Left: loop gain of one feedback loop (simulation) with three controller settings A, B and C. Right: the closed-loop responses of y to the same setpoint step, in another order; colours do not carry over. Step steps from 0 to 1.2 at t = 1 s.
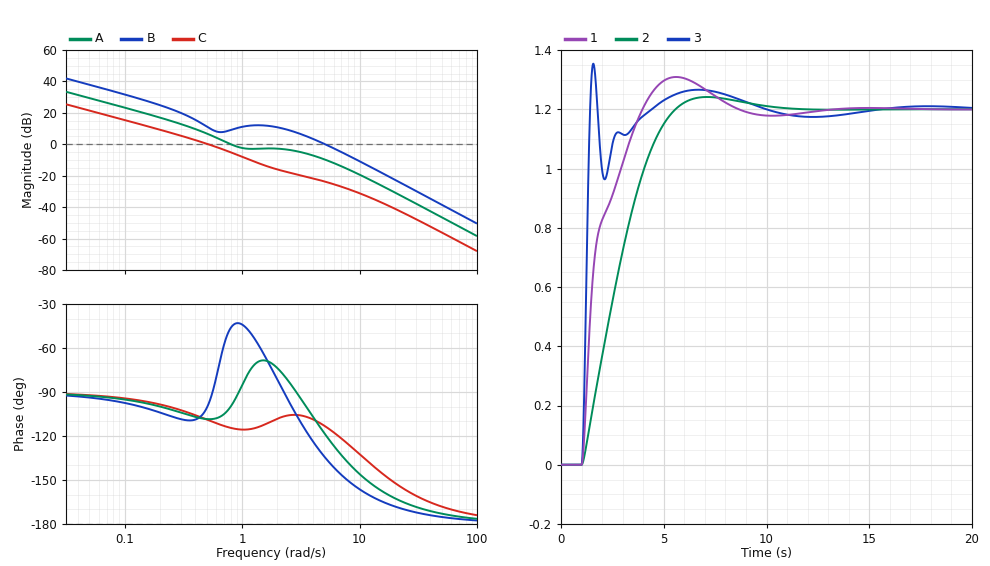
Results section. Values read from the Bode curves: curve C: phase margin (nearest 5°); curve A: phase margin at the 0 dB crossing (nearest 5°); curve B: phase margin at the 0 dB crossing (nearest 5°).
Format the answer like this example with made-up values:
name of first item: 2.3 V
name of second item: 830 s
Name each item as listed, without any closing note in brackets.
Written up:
curve C: phase margin: 70°
curve A: phase margin at the 0 dB crossing: 80°
curve B: phase margin at the 0 dB crossing: 45°
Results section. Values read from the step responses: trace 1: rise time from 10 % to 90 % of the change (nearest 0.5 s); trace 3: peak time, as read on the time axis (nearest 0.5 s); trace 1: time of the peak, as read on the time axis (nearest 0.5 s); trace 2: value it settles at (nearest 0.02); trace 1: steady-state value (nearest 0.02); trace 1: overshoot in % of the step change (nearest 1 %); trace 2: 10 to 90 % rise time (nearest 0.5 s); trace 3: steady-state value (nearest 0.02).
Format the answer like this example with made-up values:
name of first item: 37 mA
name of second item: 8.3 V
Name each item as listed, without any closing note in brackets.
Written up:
trace 1: rise time from 10 % to 90 % of the change: 2.0 s
trace 3: peak time, as read on the time axis: 1.5 s
trace 1: time of the peak, as read on the time axis: 5.5 s
trace 2: value it settles at: 1.20
trace 1: steady-state value: 1.20
trace 1: overshoot in % of the step change: 9 %
trace 2: 10 to 90 % rise time: 3.0 s
trace 3: steady-state value: 1.20
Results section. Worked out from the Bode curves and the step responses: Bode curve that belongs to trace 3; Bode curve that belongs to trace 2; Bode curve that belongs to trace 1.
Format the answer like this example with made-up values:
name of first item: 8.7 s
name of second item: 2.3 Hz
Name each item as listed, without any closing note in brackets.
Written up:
Bode curve that belongs to trace 3: B
Bode curve that belongs to trace 2: C
Bode curve that belongs to trace 1: A
